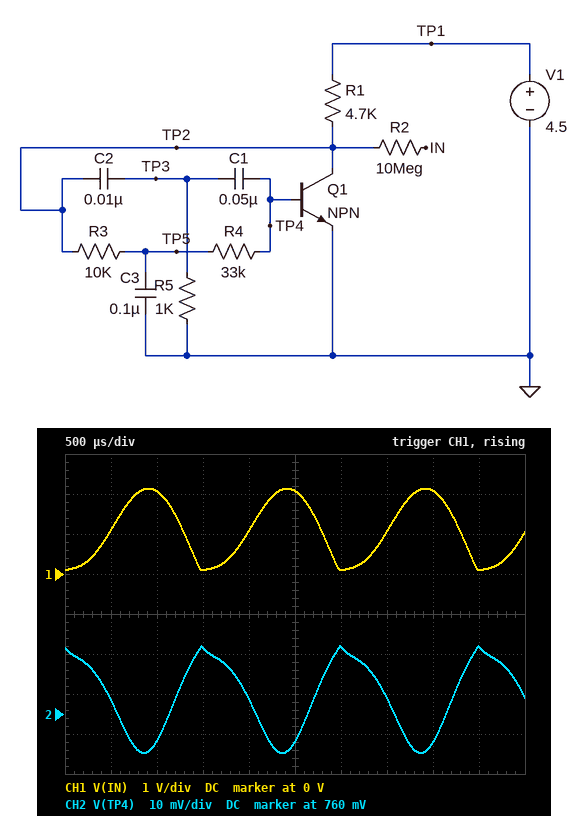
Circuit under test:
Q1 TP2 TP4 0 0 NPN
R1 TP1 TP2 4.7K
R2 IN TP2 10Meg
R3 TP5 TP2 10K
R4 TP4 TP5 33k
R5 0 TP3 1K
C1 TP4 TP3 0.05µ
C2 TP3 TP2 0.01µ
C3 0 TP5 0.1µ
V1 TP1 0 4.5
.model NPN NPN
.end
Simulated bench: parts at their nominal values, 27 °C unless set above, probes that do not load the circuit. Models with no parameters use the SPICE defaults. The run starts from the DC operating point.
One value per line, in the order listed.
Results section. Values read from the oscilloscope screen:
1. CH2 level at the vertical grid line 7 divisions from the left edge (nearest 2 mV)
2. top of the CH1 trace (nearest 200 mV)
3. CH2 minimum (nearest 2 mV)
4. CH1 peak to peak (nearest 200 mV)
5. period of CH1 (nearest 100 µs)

764 mV
2.2 V
750 mV
2.0 V
1.5 ms
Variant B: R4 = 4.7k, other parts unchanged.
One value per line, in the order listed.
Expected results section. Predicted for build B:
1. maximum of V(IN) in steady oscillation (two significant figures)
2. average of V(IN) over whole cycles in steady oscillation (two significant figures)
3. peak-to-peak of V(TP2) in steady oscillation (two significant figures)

1.9 V
950 mV
1.8 V
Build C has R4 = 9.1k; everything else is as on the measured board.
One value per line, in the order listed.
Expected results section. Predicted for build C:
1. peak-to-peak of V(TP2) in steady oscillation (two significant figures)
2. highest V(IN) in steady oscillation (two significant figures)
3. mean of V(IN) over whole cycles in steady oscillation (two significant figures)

1.9 V
2.0 V
990 mV
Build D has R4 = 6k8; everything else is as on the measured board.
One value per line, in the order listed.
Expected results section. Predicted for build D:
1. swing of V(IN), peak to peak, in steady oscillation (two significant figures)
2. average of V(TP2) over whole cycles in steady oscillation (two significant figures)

1.9 V
970 mV
